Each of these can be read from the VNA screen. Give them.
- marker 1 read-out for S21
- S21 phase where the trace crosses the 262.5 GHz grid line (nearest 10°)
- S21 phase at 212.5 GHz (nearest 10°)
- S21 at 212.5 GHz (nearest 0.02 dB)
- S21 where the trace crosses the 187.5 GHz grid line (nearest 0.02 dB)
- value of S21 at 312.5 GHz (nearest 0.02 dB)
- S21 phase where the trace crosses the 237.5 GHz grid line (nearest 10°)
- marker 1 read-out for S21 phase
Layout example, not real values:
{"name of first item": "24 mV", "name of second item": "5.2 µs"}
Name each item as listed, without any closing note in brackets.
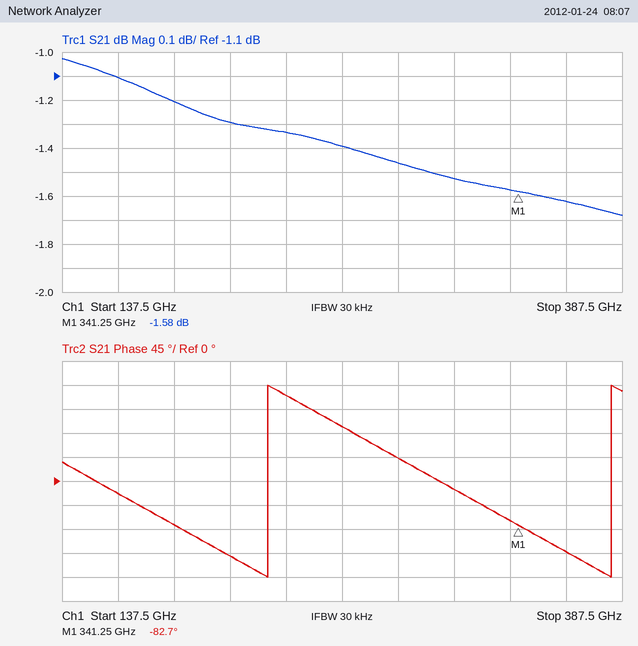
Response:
{"marker 1 read-out for S21": "-1.58 dB", "S21 phase where the trace crosses the 262.5 GHz grid line": "100°", "S21 phase at 212.5 GHz": "-140°", "S21 at 212.5 GHz": "-1.30 dB", "S21 where the trace crosses the 187.5 GHz grid line": "-1.20 dB", "value of S21 at 312.5 GHz": "-1.52 dB", "S21 phase where the trace crosses the 237.5 GHz grid line": "160°", "marker 1 read-out for S21 phase": "-82.7°"}
